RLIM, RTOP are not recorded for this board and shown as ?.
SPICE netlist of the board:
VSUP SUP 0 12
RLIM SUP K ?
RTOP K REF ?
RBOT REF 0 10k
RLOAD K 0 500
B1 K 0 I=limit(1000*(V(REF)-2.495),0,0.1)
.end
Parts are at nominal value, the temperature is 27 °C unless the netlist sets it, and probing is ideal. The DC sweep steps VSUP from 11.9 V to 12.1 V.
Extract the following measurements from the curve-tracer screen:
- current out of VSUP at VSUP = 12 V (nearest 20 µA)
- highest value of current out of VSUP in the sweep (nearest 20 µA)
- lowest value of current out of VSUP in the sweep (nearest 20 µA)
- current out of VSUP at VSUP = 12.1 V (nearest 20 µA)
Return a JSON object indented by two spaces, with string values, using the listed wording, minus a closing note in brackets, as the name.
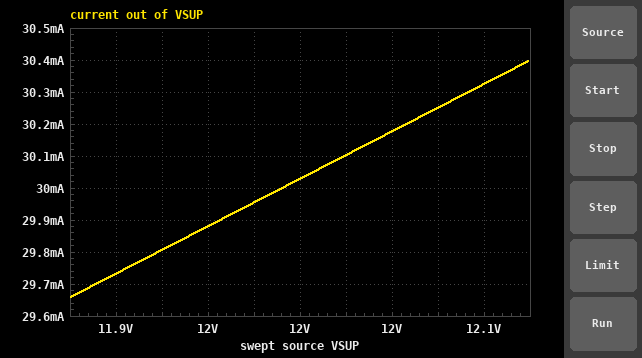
{
  "current out of VSUP at VSUP = 12 V": "29.88 mA",
  "highest value of current out of VSUP in the sweep": "30.40 mA",
  "lowest value of current out of VSUP in the sweep": "29.66 mA",
  "current out of VSUP at VSUP = 12.1 V": "30.32 mA"
}
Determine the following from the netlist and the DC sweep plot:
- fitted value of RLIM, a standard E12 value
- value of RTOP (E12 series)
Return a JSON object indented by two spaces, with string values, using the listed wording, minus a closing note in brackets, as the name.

{
  "fitted value of RLIM, a standard E12 value": "270 Ω",
  "value of RTOP": "5.6 kΩ"
}
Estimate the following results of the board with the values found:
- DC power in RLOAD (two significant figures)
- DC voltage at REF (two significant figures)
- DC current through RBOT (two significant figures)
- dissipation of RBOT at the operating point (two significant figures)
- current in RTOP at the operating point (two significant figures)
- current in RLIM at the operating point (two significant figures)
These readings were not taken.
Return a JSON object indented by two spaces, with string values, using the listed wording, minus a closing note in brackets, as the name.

{
  "DC power in RLOAD": "30 mW",
  "DC voltage at REF": "2.5 V",
  "DC current through RBOT": "250 µA",
  "dissipation of RBOT at the operating point": "620 µW",
  "current in RTOP at the operating point": "250 µA",
  "current in RLIM at the operating point": "30 mA"
}
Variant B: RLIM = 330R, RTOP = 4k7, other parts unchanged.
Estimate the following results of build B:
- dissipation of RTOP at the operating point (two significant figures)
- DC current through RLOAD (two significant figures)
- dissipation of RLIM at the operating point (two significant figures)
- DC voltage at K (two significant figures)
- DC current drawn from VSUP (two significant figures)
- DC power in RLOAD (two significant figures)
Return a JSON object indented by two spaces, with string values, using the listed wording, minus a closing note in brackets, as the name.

{
  "dissipation of RTOP at the operating point": "290 µW",
  "DC current through RLOAD": "7.3 mA",
  "dissipation of RLIM at the operating point": "210 mW",
  "DC voltage at K": "3.7 V",
  "DC current drawn from VSUP": "25 mA",
  "DC power in RLOAD": "27 mW"
}
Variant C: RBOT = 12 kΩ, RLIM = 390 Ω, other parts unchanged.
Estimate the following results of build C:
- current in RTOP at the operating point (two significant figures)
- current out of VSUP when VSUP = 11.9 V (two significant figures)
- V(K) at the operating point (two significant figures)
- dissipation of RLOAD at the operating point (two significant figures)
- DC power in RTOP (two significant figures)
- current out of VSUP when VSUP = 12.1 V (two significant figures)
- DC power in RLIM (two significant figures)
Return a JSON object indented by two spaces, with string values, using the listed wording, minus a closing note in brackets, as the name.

{
  "current in RTOP at the operating point": "210 µA",
  "current out of VSUP when VSUP = 11.9 V": "21 mA",
  "V(K) at the operating point": "3.7 V",
  "dissipation of RLOAD at the operating point": "27 mW",
  "DC power in RTOP": "240 µW",
  "current out of VSUP when VSUP = 12.1 V": "22 mA",
  "DC power in RLIM": "180 mW"
}
